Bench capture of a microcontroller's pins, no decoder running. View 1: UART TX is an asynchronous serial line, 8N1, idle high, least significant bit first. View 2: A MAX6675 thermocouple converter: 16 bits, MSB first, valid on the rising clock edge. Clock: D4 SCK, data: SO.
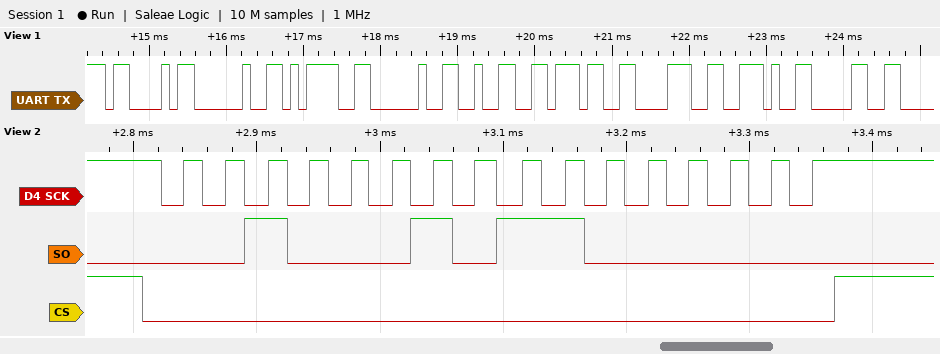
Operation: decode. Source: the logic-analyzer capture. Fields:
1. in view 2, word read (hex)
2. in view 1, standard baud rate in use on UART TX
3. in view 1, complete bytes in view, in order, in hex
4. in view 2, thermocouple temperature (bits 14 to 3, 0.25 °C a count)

0x22C0
9600 baud
0x43 0x20 0x3D 0x20 0x32 0x37 0x38 0x2E 0x30
278.00 °C
